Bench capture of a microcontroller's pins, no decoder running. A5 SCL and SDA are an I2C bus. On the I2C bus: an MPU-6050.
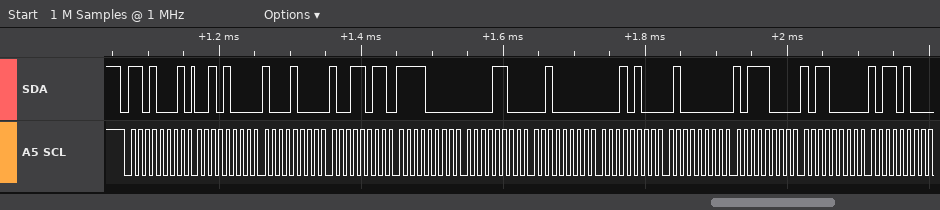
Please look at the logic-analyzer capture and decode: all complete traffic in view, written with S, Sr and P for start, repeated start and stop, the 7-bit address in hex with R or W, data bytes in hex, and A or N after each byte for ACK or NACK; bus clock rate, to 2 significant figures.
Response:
S 68R A 28 A 88 A 9B A F0 A 0C A 20 A 14 A 40 A B8 A B0 A B4 A
100 kHz
